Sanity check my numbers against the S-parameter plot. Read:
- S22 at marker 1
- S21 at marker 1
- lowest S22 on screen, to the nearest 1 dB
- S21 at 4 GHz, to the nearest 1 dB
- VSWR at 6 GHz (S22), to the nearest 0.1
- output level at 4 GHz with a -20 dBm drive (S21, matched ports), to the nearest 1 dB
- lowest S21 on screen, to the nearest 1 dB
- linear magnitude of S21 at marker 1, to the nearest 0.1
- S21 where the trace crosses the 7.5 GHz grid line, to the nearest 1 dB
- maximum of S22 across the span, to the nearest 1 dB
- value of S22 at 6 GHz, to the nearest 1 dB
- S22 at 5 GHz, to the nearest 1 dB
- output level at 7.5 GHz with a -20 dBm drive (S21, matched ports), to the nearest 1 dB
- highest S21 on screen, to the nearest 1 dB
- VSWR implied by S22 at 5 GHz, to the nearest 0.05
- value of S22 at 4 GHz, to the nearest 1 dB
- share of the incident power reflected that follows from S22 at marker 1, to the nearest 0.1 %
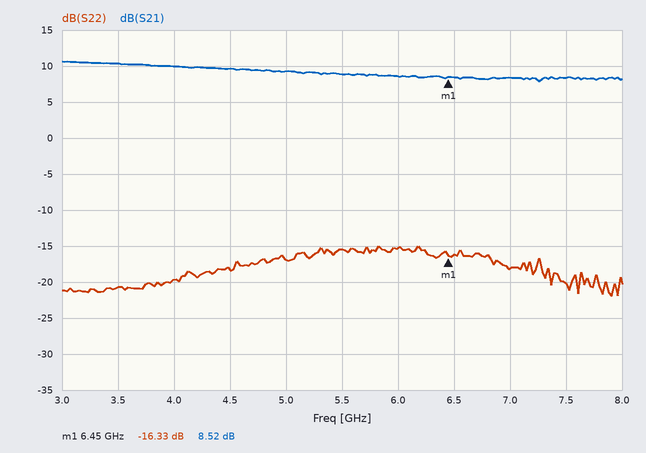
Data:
-16.33 dB
8.52 dB
-22 dB
10 dB
1.4
-10 dBm
8 dB
2.7
8 dB
-15 dB
-15 dB
-17 dB
-12 dBm
11 dB
1.35
-20 dB
2.3 %
